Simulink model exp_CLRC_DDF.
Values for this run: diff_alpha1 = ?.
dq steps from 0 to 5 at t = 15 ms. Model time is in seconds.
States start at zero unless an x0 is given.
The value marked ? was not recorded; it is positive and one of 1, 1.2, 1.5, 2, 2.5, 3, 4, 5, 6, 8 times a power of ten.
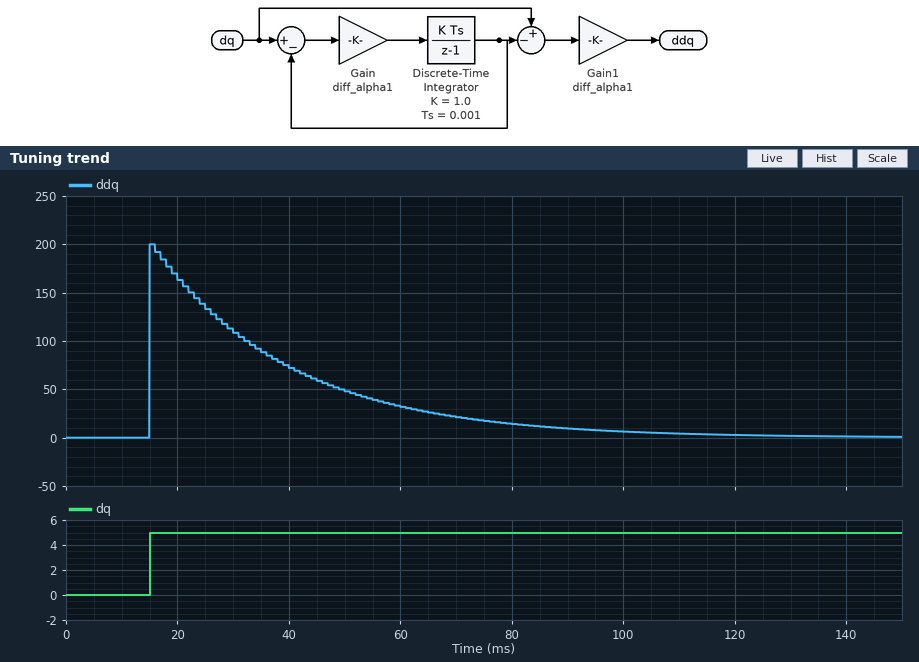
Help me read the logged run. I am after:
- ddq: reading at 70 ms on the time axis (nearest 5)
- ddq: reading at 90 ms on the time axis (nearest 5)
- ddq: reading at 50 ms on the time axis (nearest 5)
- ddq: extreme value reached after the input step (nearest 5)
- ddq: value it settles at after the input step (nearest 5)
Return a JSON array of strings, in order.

["20", "10", "50", "200", "0"]
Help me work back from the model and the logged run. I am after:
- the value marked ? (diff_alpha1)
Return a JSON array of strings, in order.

["40"]
